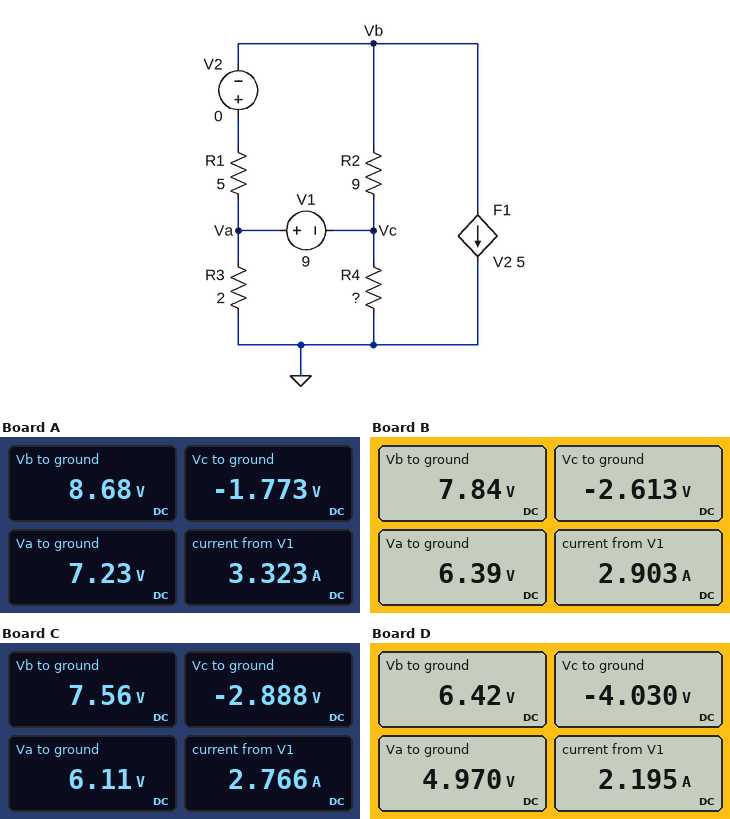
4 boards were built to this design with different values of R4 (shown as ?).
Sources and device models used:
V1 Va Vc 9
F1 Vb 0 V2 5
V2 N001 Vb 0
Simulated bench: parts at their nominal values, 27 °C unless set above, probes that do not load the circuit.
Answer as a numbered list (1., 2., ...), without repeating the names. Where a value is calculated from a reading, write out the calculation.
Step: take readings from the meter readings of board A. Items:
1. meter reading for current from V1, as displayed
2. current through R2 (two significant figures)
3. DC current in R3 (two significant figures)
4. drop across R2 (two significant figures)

1. 3.323 A
2. (8.68 V - (-1.773 V)) / 9 Ω = 1.2 A
3. (7.23 V) / 2 Ω = 3.6 A
4. 8.68 V - (-1.773 V) = 10 V
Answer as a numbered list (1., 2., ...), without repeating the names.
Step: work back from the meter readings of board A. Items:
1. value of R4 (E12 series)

1. 0.82 Ω
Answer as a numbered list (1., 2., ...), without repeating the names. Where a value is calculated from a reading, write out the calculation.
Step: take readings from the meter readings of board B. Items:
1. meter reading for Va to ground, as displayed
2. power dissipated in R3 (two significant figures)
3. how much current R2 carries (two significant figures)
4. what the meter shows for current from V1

1. 6.39 V
2. (6.39 V)^2 / 2 Ω = 20 W
3. (7.84 V - (-2.613 V)) / 9 Ω = 1.2 A
4. 2.903 A
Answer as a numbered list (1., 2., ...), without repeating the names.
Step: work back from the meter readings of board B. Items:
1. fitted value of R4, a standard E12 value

1. 1.5 Ω
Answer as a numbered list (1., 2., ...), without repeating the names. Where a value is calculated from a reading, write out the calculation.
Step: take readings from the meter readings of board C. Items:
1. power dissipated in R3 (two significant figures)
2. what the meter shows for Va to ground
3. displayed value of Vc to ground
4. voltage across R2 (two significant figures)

1. (6.11 V)^2 / 2 Ω = 19 W
2. 6.11 V
3. -2.888 V
4. 7.56 V - (-2.888 V) = 10 V
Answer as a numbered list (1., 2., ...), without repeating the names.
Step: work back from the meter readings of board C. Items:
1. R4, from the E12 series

1. 1.8 Ω
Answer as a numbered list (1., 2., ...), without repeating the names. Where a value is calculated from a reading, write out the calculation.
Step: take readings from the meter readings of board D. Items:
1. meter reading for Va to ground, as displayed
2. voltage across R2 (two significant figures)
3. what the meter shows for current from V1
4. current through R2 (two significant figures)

1. 4.970 V
2. 6.42 V - (-4.03 V) = 10 V
3. 2.195 A
4. (6.42 V - (-4.03 V)) / 9 Ω = 1.2 A
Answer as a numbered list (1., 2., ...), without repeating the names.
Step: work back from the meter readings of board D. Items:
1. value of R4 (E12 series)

1. 3.9 Ω
